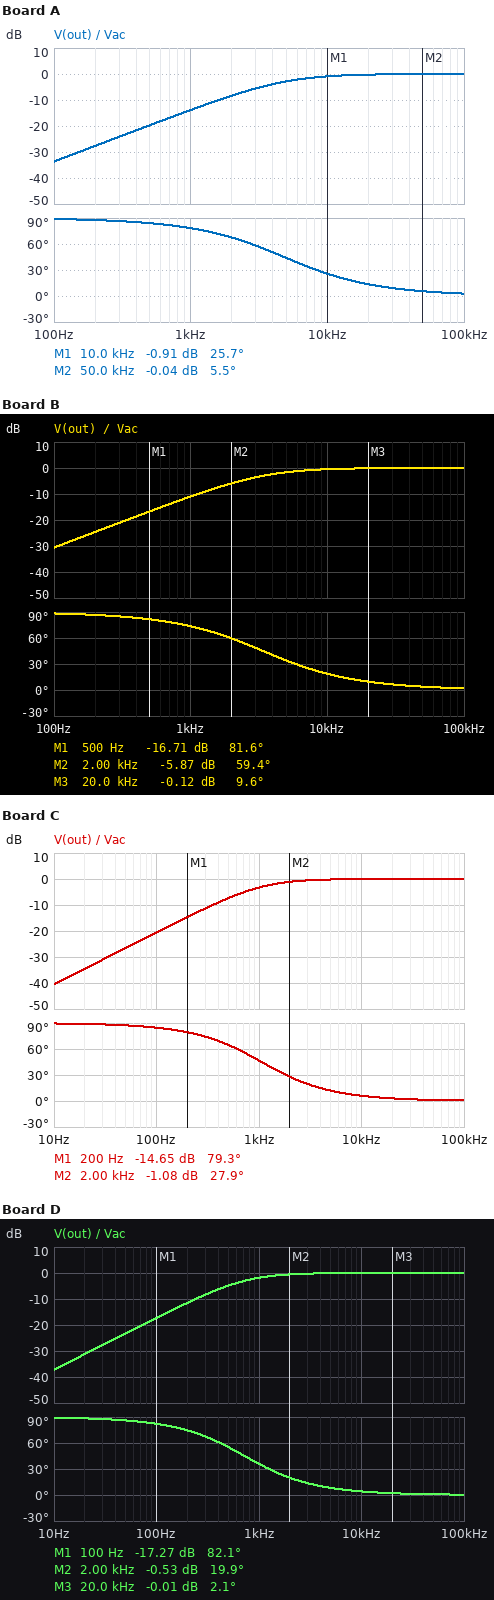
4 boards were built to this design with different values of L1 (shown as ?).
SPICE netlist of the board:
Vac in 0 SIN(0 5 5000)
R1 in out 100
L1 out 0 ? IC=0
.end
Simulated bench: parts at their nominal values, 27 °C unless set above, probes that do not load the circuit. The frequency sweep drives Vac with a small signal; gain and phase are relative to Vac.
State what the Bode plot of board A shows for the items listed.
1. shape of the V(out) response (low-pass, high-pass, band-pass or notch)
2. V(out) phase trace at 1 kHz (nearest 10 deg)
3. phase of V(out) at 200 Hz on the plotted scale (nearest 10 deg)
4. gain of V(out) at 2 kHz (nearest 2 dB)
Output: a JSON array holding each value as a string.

["high-pass", "80 deg", "90 deg", "-8 dB"]
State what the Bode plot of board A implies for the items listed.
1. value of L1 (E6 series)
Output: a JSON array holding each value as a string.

["3.3 mH"]
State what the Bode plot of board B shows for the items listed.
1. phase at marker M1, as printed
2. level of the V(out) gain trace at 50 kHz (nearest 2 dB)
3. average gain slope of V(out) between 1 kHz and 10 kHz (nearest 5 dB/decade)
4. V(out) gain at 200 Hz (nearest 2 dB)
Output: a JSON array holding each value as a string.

["81.6 deg", "0 dB", "10 dB/decade", "-24 dB"]
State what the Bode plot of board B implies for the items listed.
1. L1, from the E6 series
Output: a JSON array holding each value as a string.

["4.7 mH"]
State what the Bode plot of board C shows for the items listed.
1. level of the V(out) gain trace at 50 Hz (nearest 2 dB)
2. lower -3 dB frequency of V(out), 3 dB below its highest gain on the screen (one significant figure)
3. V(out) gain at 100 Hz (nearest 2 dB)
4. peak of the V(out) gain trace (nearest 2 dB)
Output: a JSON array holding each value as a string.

["-26 dB", "1 kHz", "-20 dB", "0 dB"]
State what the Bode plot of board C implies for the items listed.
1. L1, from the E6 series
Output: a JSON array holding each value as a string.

["15 mH"]
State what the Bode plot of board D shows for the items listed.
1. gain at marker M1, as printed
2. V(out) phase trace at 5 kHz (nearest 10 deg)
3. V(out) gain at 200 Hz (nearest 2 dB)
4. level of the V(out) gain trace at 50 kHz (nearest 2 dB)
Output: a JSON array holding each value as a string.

["-17.27 dB", "10 deg", "-12 dB", "0 dB"]
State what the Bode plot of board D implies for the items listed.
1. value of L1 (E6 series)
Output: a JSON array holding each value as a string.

["22 mH"]
